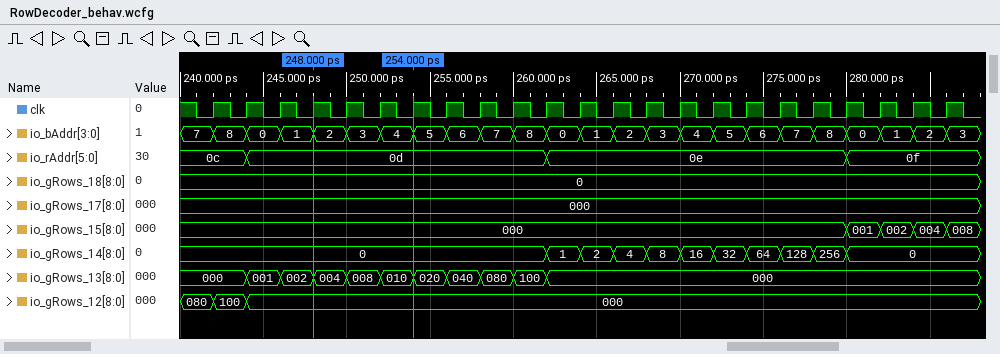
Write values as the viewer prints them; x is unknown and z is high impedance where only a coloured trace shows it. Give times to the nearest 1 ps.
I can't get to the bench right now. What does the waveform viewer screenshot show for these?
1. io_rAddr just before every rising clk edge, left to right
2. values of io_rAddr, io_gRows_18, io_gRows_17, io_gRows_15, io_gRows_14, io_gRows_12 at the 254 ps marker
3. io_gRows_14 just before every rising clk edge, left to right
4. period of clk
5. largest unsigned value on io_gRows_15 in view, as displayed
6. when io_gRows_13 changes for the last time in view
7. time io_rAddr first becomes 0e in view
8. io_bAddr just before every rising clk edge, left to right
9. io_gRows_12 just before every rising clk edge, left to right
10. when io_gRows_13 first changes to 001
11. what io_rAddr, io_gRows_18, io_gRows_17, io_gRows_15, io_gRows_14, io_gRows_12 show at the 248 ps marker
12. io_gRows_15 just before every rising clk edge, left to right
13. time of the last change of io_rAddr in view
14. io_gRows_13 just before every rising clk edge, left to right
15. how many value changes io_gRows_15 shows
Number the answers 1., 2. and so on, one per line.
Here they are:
1. 0c, 0c, 0d, 0d, 0d, 0d, 0d, 0d, 0d, 0d, 0d, 0e, 0e, 0e, 0e, 0e, 0e, 0e, 0e, 0e, 0f, 0f, 0f
2. io_rAddr=0d, io_gRows_18=0, io_gRows_17=000, io_gRows_15=000, io_gRows_14=0, io_gRows_12=000
3. 0, 0, 0, 0, 0, 0, 0, 0, 0, 0, 0, 1, 2, 4, 8, 16, 32, 64, 128, 256, 0, 0, 0
4. 2 ps
5. 008
6. 262 ps
7. 262 ps
8. 7, 8, 0, 1, 2, 3, 4, 5, 6, 7, 8, 0, 1, 2, 3, 4, 5, 6, 7, 8, 0, 1, 2
9. 080, 100, 000, 000, 000, 000, 000, 000, 000, 000, 000, 000, 000, 000, 000, 000, 000, 000, 000, 000, 000, 000, 000
10. 244 ps
11. io_rAddr=0d, io_gRows_18=0, io_gRows_17=000, io_gRows_15=000, io_gRows_14=0, io_gRows_12=000
12. 000, 000, 000, 000, 000, 000, 000, 000, 000, 000, 000, 000, 000, 000, 000, 000, 000, 000, 000, 000, 001, 002, 004
13. 280 ps
14. 000, 000, 001, 002, 004, 008, 010, 020, 040, 080, 100, 000, 000, 000, 000, 000, 000, 000, 000, 000, 000, 000, 000
15. 4
